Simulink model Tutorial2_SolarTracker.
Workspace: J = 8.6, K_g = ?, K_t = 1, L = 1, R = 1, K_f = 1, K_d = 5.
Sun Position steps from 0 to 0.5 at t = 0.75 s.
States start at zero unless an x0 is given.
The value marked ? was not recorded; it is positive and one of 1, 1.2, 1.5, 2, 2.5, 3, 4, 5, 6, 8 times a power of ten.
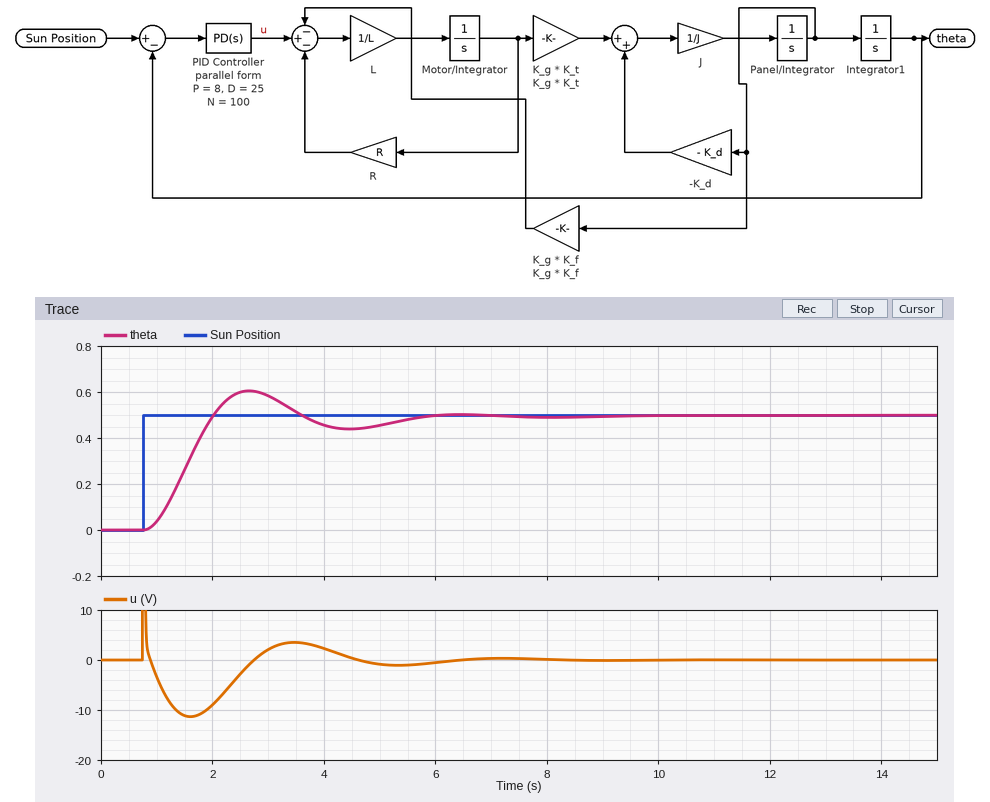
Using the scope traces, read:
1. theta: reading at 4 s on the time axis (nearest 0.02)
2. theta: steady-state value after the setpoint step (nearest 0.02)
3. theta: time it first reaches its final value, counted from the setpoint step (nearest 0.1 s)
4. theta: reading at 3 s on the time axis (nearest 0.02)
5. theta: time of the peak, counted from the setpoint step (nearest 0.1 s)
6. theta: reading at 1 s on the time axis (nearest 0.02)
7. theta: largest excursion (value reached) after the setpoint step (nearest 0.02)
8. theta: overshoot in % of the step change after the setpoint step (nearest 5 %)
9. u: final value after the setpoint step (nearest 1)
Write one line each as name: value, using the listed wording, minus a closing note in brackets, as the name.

theta: reading at 4 s on the time axis: 0.46
theta: steady-state value after the setpoint step: 0.50
theta: time it first reaches its final value, counted from the setpoint step: 1.3 s
theta: reading at 3 s on the time axis: 0.58
theta: time of the peak, counted from the setpoint step: 1.9 s
theta: reading at 1 s on the time axis: 0.04
theta: largest excursion (value reached) after the setpoint step: 0.60
theta: overshoot in % of the step change after the setpoint step: 20 %
u: final value after the setpoint step: 0
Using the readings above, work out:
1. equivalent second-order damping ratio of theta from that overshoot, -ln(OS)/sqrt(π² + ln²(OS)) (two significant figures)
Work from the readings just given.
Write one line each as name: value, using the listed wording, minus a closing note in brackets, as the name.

equivalent second-order damping ratio of theta from that overshoot, -ln(OS)/sqrt(π² + ln²(OS)): 0.46
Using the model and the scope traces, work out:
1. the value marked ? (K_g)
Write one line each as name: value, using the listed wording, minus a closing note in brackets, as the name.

the value marked ?: 1
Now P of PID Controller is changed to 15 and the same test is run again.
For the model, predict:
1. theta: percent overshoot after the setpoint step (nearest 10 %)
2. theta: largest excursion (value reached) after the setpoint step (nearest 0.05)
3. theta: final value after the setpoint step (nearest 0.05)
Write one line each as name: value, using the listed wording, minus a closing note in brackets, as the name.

theta: percent overshoot after the setpoint step: 40 %
theta: largest excursion (value reached) after the setpoint step: 0.70
theta: final value after the setpoint step: 0.50
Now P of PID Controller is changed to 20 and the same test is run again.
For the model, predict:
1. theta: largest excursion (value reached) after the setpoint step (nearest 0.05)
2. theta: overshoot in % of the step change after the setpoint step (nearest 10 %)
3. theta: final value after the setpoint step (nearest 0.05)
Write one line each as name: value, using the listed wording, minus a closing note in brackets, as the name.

theta: largest excursion (value reached) after the setpoint step: 0.75
theta: overshoot in % of the step change after the setpoint step: 50 %
theta: final value after the setpoint step: 0.50
